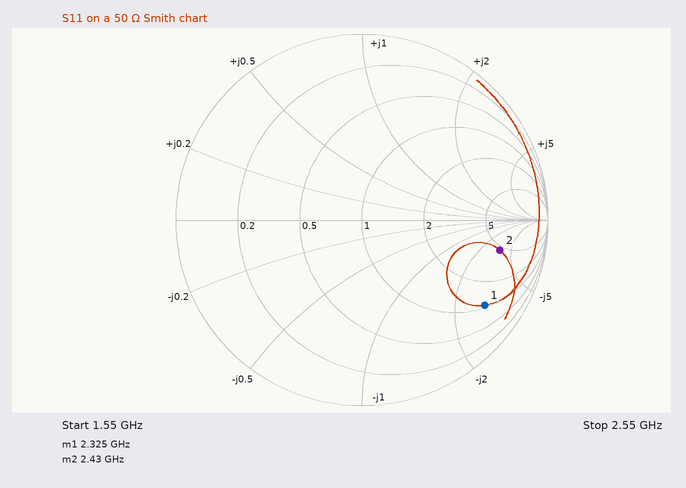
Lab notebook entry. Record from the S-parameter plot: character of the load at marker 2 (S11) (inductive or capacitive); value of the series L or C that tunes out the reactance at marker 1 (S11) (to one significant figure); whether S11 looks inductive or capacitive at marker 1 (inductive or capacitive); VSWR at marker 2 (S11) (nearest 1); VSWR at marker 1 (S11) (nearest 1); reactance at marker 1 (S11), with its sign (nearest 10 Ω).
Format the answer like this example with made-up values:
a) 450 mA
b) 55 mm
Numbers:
a) capacitive
b) 10 nH
c) capacitive
d) 7
e) 9
f) -140 Ω
